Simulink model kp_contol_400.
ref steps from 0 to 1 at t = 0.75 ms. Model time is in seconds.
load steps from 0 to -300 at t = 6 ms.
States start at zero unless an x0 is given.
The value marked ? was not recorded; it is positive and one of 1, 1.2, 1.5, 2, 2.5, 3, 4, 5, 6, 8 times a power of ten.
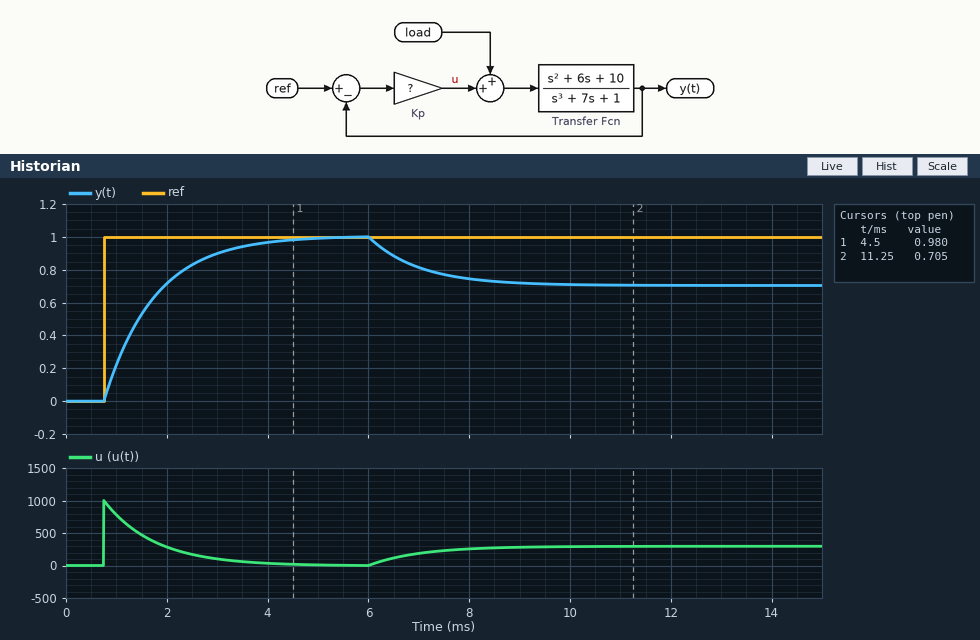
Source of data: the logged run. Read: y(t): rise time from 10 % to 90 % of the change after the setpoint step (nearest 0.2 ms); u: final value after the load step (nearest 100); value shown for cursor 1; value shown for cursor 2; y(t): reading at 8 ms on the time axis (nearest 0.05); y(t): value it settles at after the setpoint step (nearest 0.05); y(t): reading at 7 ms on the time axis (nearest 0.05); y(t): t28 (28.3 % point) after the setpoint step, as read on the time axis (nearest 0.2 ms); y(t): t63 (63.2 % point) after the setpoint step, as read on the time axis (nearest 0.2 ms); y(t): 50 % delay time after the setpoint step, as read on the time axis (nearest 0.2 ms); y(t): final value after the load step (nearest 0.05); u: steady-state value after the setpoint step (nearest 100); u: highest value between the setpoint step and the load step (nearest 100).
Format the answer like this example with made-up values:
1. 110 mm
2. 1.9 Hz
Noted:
1. 2.2 ms
2. 300
3. 0.980
4. 0.705
5. 0.75
6. 1.00
7. 0.80
8. 1.0 ms
9. 1.8 ms
10. 1.4 ms
11. 0.70
12. 0
13. 1000
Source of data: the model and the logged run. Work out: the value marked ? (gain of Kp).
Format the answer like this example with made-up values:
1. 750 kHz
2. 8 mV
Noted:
1. 1000
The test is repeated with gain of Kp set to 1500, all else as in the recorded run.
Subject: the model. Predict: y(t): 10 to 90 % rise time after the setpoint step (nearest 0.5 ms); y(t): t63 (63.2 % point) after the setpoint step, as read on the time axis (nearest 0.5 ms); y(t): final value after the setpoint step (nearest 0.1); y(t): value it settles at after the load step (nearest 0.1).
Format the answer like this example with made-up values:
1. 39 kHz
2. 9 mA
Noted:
1. 1.5 ms
2. 1.5 ms
3. 1.0
4. 0.8
